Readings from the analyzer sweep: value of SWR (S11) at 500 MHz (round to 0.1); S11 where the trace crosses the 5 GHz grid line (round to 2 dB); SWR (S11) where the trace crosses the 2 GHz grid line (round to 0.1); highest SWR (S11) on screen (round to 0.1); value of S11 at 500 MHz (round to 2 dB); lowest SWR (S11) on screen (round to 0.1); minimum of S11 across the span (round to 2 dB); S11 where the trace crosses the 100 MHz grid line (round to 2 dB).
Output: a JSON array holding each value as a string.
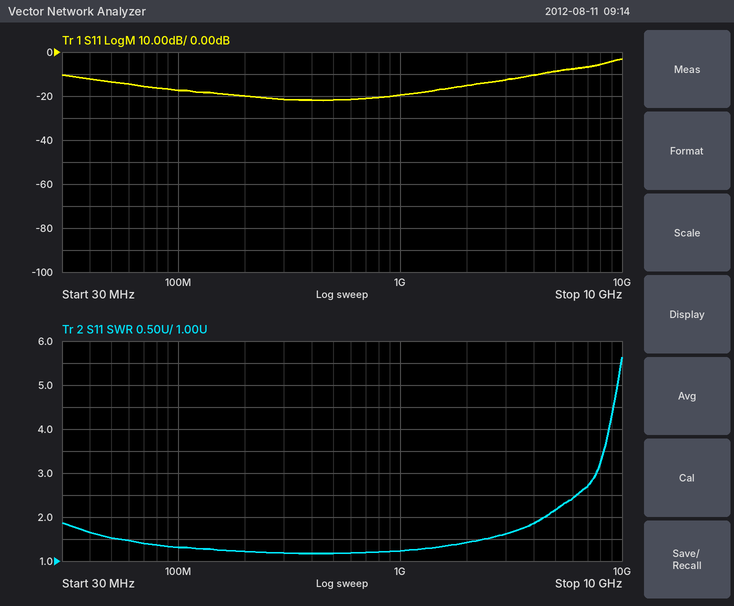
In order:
["1.2", "-8 dB", "1.4", "5.6", "-22 dB", "1.2", "-22 dB", "-18 dB"]
